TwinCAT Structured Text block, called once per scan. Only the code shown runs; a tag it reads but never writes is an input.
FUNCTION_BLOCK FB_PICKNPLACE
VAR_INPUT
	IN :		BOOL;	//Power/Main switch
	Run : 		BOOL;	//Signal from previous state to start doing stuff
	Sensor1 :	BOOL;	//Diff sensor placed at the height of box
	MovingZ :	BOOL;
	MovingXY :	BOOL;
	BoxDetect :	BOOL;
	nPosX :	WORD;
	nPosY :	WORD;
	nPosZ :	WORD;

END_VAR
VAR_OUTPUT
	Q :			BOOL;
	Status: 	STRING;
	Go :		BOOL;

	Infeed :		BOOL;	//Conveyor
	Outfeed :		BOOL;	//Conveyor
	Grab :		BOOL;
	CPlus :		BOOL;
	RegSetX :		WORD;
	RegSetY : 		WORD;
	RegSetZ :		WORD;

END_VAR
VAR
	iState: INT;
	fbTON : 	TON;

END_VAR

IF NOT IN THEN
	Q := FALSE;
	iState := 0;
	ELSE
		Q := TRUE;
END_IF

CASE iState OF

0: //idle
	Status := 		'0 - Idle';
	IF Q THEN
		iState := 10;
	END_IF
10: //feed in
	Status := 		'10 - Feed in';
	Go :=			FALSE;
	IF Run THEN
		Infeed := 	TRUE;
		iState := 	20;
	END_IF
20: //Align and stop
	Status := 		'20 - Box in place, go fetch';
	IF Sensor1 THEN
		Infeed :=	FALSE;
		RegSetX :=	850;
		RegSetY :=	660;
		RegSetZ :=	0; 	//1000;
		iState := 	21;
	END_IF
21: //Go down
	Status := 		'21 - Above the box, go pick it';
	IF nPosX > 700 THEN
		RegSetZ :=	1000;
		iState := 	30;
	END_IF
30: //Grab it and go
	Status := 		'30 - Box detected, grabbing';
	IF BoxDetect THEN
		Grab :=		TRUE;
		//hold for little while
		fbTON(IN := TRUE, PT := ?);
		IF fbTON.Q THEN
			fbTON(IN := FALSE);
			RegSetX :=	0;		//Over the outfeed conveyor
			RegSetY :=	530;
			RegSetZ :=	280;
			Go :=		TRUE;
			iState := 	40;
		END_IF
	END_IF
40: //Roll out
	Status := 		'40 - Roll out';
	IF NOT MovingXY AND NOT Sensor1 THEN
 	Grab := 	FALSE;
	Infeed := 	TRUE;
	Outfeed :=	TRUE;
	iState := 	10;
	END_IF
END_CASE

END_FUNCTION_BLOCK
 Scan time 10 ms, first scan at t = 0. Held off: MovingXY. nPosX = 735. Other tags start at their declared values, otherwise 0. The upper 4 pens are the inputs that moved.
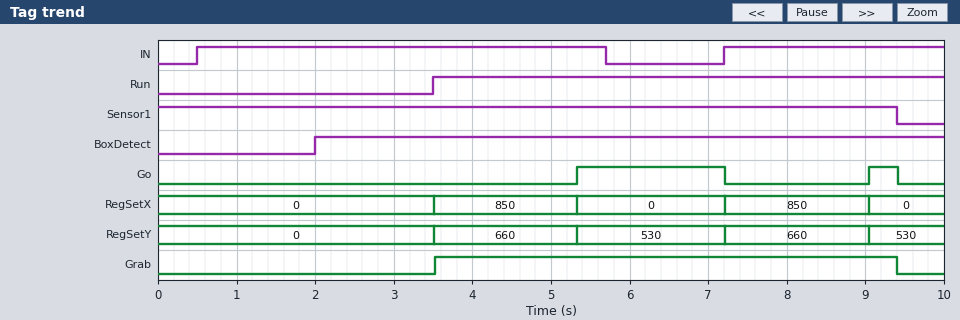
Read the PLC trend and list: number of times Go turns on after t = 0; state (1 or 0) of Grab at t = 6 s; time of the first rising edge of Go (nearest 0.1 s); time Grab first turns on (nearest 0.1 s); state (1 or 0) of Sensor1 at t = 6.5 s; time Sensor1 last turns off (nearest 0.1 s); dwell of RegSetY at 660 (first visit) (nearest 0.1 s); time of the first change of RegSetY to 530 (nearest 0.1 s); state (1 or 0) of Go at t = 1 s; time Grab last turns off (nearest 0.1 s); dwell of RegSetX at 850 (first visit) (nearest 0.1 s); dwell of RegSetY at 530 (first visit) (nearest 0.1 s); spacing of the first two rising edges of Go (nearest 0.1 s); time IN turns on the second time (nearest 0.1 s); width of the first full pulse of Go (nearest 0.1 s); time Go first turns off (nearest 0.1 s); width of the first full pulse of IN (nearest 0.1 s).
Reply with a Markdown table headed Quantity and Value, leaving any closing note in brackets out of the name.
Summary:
| Quantity | Value |
|---|---|
| number of times Go turns on after t = 0 | 2 |
| state (1 or 0) of Grab at t = 6 s | 1 |
| time of the first rising edge of Go | 5.3 s |
| time Grab first turns on | 3.5 s |
| state (1 or 0) of Sensor1 at t = 6.5 s | 1 |
| time Sensor1 last turns off | 9.4 s |
| dwell of RegSetY at 660 (first visit) | 1.8 s |
| time of the first change of RegSetY to 530 | 5.3 s |
| state (1 or 0) of Go at t = 1 s | 0 |
| time Grab last turns off | 9.4 s |
| dwell of RegSetX at 850 (first visit) | 1.8 s |
| dwell of RegSetY at 530 (first visit) | 1.9 s |
| spacing of the first two rising edges of Go | 3.7 s |
| time IN turns on the second time | 7.2 s |
| width of the first full pulse of Go | 1.9 s |
| time Go first turns off | 7.2 s |
| width of the first full pulse of IN | 5.2 s |
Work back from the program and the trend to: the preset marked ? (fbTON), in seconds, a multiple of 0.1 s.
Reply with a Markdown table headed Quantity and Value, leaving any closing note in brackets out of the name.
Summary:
| Quantity | Value |
|---|---|
| the preset marked ? (fbTON), in seconds, a multiple of 0.1 s | 1.8 s |
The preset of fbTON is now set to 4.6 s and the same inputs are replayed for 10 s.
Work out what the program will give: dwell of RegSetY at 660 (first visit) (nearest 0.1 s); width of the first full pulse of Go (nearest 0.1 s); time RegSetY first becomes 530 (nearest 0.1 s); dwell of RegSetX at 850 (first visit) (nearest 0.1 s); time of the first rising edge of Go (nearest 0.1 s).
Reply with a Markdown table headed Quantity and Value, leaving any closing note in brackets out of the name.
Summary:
| Quantity | Value |
|---|---|
| dwell of RegSetY at 660 (first visit) | 4.6 s |
| width of the first full pulse of Go | 1.3 s |
| time RegSetY first becomes 530 | 8.1 s |
| dwell of RegSetX at 850 (first visit) | 4.6 s |
| time of the first rising edge of Go | 8.1 s |
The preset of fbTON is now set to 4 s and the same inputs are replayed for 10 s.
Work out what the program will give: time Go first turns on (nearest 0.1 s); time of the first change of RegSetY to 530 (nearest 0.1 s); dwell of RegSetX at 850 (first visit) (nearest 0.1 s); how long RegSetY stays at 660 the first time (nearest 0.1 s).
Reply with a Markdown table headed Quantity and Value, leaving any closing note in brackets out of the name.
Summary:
| Quantity | Value |
|---|---|
| time Go first turns on | 7.5 s |
| time of the first change of RegSetY to 530 | 7.5 s |
| dwell of RegSetX at 850 (first visit) | 4.0 s |
| how long RegSetY stays at 660 the first time | 4.0 s |
